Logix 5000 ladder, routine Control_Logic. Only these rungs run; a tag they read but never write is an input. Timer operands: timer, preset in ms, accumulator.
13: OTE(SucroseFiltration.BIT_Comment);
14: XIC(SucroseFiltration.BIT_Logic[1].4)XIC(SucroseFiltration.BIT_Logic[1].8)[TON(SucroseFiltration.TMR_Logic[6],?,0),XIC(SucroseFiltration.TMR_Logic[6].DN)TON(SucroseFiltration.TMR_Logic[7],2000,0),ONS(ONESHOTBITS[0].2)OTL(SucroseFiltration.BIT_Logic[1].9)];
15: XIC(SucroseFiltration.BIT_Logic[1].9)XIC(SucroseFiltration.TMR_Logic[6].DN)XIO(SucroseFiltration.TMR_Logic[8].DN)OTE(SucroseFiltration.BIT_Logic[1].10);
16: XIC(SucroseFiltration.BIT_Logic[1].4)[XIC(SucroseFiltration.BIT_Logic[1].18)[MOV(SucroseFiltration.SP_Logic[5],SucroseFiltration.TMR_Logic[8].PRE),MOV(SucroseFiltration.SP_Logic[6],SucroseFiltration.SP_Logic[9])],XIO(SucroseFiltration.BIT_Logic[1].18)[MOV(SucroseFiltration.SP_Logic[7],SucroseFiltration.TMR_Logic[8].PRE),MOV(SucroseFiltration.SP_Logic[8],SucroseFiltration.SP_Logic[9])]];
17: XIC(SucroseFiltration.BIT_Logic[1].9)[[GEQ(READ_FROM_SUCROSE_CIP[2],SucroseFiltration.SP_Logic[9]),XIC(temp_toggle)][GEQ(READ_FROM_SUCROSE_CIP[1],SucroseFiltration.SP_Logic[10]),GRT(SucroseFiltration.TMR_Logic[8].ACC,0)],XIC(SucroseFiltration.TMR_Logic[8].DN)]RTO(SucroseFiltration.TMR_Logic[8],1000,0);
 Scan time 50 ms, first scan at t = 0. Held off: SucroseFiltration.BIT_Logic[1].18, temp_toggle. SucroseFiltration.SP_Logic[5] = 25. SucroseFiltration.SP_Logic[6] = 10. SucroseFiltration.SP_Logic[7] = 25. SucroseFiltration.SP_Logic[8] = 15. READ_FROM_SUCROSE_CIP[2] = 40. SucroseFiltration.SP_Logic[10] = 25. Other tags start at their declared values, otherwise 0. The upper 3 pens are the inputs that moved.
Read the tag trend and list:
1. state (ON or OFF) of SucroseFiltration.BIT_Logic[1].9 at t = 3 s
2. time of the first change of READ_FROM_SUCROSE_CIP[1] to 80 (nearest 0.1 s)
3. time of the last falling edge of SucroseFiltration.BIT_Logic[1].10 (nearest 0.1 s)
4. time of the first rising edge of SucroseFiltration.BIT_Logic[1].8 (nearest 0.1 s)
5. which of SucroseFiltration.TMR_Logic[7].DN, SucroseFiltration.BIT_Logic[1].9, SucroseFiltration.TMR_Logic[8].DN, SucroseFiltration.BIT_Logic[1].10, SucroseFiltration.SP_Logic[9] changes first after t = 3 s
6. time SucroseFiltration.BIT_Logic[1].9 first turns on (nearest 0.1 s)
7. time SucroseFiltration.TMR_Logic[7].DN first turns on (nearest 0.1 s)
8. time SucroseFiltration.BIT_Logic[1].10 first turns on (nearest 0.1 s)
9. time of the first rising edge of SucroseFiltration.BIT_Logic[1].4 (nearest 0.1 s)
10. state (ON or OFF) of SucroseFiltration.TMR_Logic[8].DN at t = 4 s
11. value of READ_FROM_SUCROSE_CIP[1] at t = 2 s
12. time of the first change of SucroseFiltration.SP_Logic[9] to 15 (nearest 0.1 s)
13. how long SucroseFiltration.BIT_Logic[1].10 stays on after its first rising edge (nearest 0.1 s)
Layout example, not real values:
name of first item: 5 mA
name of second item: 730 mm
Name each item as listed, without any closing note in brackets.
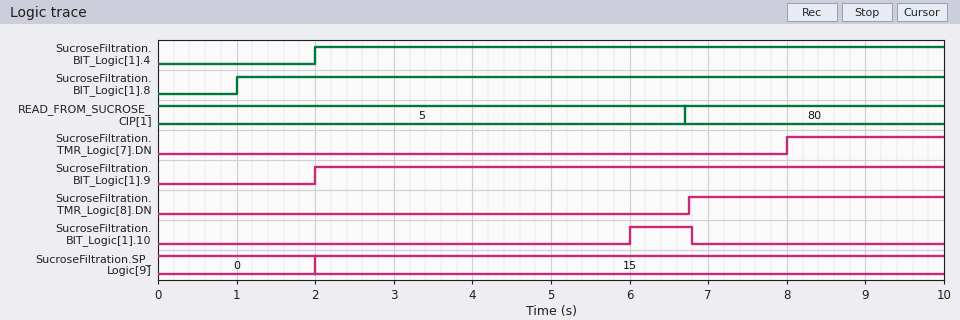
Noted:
state (ON or OFF) of SucroseFiltration.BIT_Logic[1].9 at t = 3 s: ON
time of the first change of READ_FROM_SUCROSE_CIP[1] to 80: 6.7 s
time of the last falling edge of SucroseFiltration.BIT_Logic[1].10: 6.8 s
time of the first rising edge of SucroseFiltration.BIT_Logic[1].8: 1.0 s
which of SucroseFiltration.TMR_Logic[7].DN, SucroseFiltration.BIT_Logic[1].9, SucroseFiltration.TMR_Logic[8].DN, SucroseFiltration.BIT_Logic[1].10, SucroseFiltration.SP_Logic[9] changes first after t = 3 s: SucroseFiltration.BIT_Logic[1].10
time SucroseFiltration.BIT_Logic[1].9 first turns on: 2.0 s
time SucroseFiltration.TMR_Logic[7].DN first turns on: 8.0 s
time SucroseFiltration.BIT_Logic[1].10 first turns on: 6.0 s
time of the first rising edge of SucroseFiltration.BIT_Logic[1].4: 2.0 s
state (ON or OFF) of SucroseFiltration.TMR_Logic[8].DN at t = 4 s: OFF
value of READ_FROM_SUCROSE_CIP[1] at t = 2 s: 5
time of the first change of SucroseFiltration.SP_Logic[9] to 15: 2.0 s
how long SucroseFiltration.BIT_Logic[1].10 stays on after its first rising edge: 0.8 s
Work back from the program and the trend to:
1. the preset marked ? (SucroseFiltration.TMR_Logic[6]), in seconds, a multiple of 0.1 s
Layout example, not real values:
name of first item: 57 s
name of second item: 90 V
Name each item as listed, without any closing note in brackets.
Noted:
the preset marked ? (SucroseFiltration.TMR_Logic[6]), in seconds, a multiple of 0.1 s: 4.0 s
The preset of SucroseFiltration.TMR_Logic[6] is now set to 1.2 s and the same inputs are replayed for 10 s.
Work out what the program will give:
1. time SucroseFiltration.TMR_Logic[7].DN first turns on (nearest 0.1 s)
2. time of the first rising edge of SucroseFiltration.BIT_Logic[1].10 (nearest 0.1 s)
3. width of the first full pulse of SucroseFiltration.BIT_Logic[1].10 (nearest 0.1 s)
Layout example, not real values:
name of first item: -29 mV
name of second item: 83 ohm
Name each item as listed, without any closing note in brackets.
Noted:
time SucroseFiltration.TMR_Logic[7].DN first turns on: 5.2 s
time of the first rising edge of SucroseFiltration.BIT_Logic[1].10: 3.2 s
width of the first full pulse of SucroseFiltration.BIT_Logic[1].10: 3.6 s
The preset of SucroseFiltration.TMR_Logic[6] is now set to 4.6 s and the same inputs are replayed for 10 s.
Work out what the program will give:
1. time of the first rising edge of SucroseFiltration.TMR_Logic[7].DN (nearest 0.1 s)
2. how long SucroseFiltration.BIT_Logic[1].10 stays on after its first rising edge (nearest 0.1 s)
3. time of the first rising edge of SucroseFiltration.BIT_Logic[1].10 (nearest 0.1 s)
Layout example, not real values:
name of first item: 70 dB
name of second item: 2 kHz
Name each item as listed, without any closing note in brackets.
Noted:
time of the first rising edge of SucroseFiltration.TMR_Logic[7].DN: 8.6 s
how long SucroseFiltration.BIT_Logic[1].10 stays on after its first rising edge: 0.2 s
time of the first rising edge of SucroseFiltration.BIT_Logic[1].10: 6.6 s
